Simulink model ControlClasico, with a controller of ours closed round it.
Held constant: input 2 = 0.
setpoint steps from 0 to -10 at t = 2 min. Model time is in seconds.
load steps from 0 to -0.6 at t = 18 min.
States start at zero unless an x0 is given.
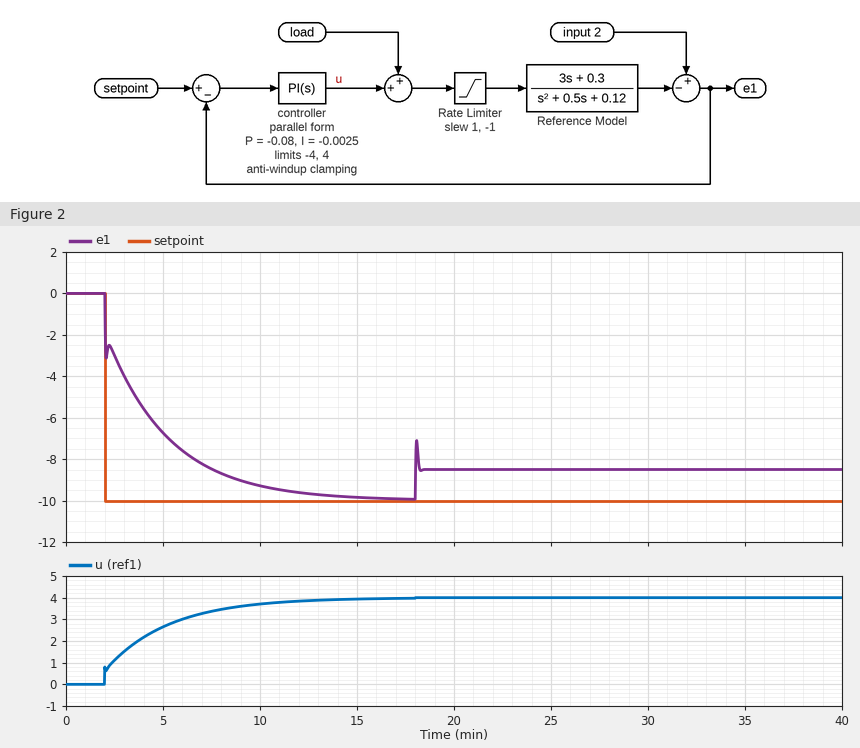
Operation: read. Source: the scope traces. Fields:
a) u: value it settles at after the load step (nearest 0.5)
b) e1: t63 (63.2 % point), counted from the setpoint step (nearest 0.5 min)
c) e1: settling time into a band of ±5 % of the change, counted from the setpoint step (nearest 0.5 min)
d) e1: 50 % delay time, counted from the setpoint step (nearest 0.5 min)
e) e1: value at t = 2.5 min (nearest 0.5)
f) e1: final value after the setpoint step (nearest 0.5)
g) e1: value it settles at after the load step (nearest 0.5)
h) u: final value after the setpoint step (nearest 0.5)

4.0
2.5 min
9.0 min
1.5 min
-3.0
-10.0
-8.5
4.0
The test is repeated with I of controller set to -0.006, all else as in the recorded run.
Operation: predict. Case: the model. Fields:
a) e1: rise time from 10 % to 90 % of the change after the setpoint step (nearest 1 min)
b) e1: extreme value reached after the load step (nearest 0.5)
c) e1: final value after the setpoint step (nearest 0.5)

3 min
-7.0
-10.0
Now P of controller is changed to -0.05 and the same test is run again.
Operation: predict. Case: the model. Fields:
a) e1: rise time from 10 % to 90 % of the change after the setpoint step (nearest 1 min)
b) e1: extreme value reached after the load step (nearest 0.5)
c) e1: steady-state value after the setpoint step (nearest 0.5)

7 min
-7.0
-10.0
